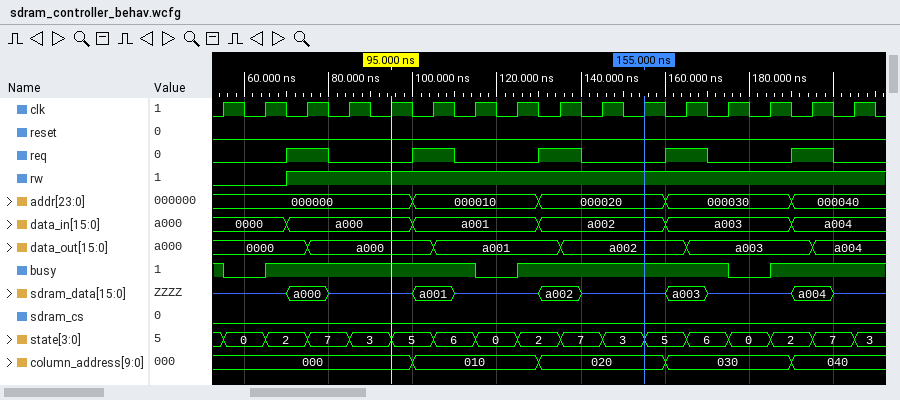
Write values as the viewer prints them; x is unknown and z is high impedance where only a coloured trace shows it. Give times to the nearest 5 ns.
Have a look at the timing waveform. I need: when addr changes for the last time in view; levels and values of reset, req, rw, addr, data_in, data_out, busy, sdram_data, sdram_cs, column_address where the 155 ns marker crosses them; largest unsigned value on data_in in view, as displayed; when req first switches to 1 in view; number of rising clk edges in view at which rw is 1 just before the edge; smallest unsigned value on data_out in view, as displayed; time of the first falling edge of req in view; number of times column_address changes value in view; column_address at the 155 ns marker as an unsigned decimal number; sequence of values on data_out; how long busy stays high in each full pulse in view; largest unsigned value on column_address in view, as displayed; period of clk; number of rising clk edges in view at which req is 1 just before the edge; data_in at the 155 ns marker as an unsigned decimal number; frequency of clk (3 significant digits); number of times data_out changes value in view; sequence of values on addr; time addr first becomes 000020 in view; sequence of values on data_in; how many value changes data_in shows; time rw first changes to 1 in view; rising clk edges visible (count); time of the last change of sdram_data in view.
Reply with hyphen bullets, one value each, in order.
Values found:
- 190 ns
- reset=0, req=0, rw=1, addr=000020, data_in=a002, data_out=a002, busy=1, sdram_data=z, sdram_cs=0, column_address=020
- a004
- 70 ns
- 14
- 0000
- 80 ns
- 4
- 32
- 0000, a000, a001, a002, a003, a004
- 50 ns, 50 ns
- 040
- 10 ns
- 5
- 40962
- 100 MHz
- 5
- 000000, 000010, 000020, 000030, 000040
- 130 ns
- 0000, a000, a001, a002, a003, a004
- 5
- 70 ns
- 16
- 200 ns
